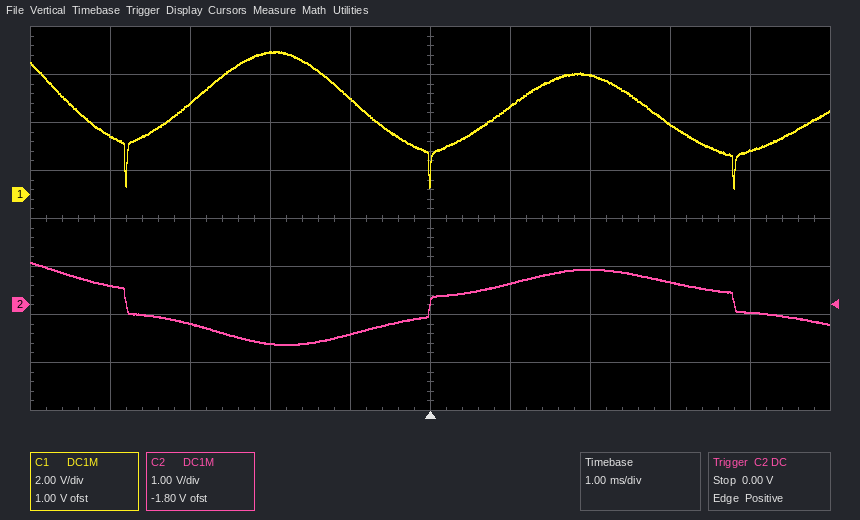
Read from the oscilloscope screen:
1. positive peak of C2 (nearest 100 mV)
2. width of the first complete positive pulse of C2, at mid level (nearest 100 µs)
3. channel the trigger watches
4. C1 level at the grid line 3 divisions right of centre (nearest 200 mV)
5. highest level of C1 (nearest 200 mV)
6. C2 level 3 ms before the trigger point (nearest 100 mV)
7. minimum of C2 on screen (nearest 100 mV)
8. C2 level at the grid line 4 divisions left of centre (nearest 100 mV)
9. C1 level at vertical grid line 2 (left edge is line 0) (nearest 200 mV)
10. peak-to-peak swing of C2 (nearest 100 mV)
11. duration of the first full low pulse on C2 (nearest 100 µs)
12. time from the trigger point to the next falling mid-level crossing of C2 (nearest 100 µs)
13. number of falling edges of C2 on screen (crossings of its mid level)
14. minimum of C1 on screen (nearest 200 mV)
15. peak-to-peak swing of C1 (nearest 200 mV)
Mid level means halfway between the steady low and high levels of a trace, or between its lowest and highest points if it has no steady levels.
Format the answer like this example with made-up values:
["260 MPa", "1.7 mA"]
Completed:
["900 mV", "3.8 ms", "C2", "3.0 V", "6.0 V", "-400 mV", "-800 mV", "400 mV", "3.8 V", "1.7 V", "3.8 ms", "3.8 ms", "2", "200 mV", "5.8 V"]
